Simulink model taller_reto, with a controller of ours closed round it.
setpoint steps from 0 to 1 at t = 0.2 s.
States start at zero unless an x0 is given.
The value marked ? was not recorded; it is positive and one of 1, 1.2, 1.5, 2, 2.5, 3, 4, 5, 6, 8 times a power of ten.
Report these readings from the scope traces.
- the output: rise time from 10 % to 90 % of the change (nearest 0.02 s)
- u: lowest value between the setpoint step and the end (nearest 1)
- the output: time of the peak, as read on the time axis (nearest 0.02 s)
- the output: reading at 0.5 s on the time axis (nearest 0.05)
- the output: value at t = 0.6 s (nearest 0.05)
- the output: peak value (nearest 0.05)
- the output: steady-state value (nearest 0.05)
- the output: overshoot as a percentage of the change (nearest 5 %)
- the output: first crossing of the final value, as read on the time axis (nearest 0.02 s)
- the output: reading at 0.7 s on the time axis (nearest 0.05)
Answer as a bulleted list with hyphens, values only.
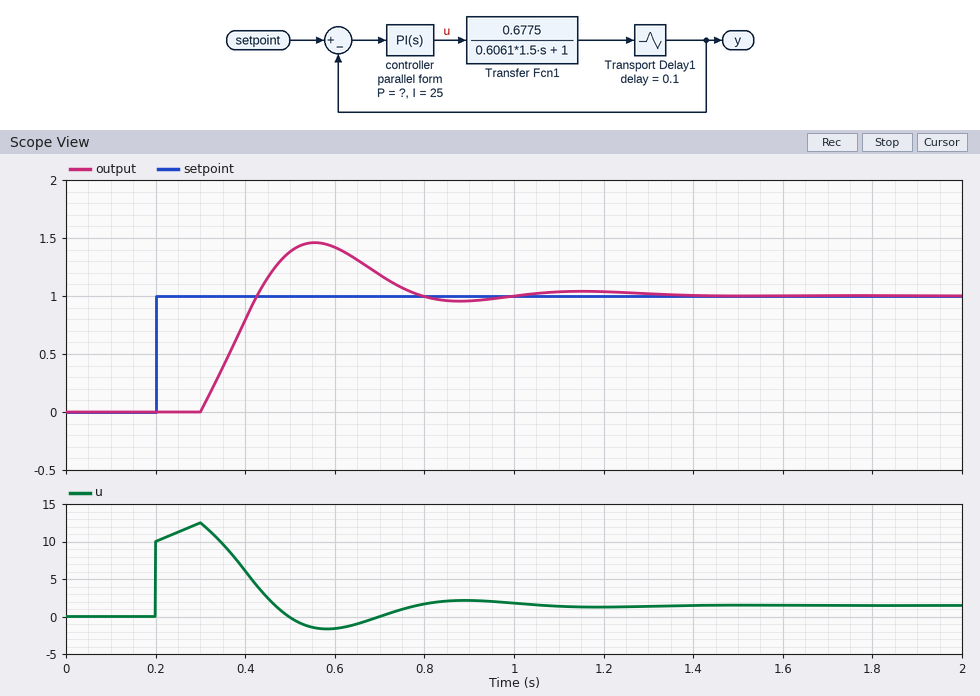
- 0.10 s
- -2
- 0.56 s
- 1.40
- 1.40
- 1.45
- 1.00
- 45 %
- 0.42 s
- 1.20
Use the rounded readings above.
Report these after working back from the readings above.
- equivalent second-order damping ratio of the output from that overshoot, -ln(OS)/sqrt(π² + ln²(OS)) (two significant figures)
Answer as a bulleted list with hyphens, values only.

- 0.25
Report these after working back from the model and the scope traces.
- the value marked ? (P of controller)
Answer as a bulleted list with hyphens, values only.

- 10
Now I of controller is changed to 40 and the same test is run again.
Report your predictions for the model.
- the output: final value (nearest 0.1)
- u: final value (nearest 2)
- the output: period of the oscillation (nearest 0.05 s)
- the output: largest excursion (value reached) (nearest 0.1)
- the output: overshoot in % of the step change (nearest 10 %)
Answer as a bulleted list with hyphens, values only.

- 1.0
- 2
- 0.65 s
- 1.7
- 70 %
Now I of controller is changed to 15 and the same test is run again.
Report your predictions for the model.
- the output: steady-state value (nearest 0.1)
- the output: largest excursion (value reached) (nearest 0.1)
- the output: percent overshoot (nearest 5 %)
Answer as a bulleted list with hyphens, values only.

- 1.0
- 1.3
- 30 %
